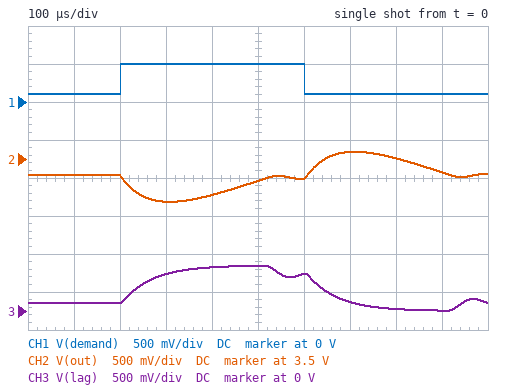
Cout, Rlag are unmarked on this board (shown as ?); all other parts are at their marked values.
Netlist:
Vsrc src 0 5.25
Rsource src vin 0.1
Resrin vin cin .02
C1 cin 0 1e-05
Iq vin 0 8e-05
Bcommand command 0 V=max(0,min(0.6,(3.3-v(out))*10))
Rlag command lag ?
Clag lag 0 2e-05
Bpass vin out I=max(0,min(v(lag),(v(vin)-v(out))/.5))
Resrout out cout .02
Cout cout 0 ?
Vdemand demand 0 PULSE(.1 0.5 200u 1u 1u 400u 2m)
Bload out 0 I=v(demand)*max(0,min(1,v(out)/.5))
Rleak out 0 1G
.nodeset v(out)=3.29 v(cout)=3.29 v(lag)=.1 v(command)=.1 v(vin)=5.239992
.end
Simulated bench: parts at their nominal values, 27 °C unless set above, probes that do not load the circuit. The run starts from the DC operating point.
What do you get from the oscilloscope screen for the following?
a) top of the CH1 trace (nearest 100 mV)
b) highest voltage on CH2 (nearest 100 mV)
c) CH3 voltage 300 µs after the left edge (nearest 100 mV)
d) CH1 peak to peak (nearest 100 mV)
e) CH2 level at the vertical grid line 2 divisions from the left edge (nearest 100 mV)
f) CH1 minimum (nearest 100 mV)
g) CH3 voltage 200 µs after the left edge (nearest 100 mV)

500 mV
3.6 V
500 mV
400 mV
3.3 V
100 mV
100 mV
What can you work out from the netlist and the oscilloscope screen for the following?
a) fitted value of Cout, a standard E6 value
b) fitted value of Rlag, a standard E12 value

47 µF
3.3 Ω
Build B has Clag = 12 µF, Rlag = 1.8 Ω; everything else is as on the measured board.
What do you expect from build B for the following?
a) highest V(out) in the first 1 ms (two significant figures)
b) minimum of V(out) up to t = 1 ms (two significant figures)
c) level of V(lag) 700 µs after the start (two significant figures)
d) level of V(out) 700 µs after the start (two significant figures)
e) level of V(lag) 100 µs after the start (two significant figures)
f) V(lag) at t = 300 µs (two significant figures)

3.4 V
3.2 V
18 mV
3.3 V
100 mV
580 mV
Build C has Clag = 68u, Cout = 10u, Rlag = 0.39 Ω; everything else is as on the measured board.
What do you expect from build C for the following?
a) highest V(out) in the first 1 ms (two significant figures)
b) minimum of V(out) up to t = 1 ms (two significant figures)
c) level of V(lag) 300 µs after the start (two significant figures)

3.9 V
2.6 V
590 mV
